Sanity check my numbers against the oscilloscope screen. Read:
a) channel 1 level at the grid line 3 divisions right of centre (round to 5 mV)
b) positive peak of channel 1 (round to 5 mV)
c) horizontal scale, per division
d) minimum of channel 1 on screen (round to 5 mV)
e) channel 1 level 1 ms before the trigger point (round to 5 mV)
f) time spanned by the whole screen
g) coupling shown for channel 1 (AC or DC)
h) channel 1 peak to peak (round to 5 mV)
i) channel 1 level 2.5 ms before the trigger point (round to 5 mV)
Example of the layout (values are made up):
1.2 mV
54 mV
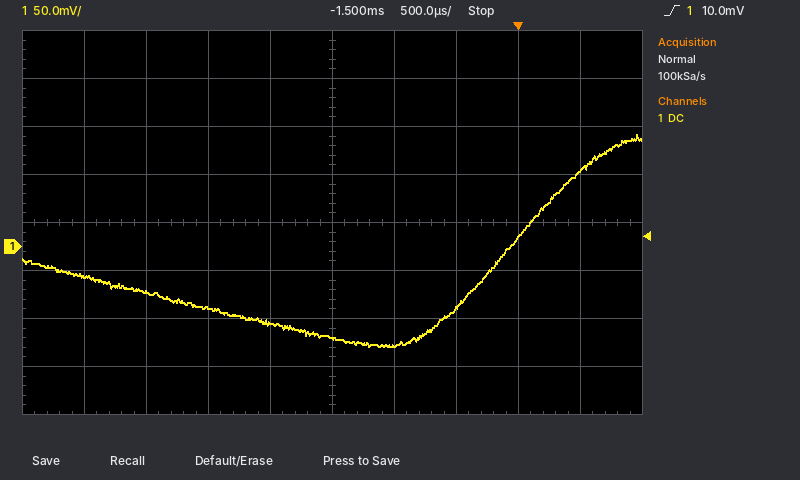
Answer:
10 mV
115 mV
500 µs
-105 mV
-105 mV
5 ms
DC
220 mV
-65 mV
